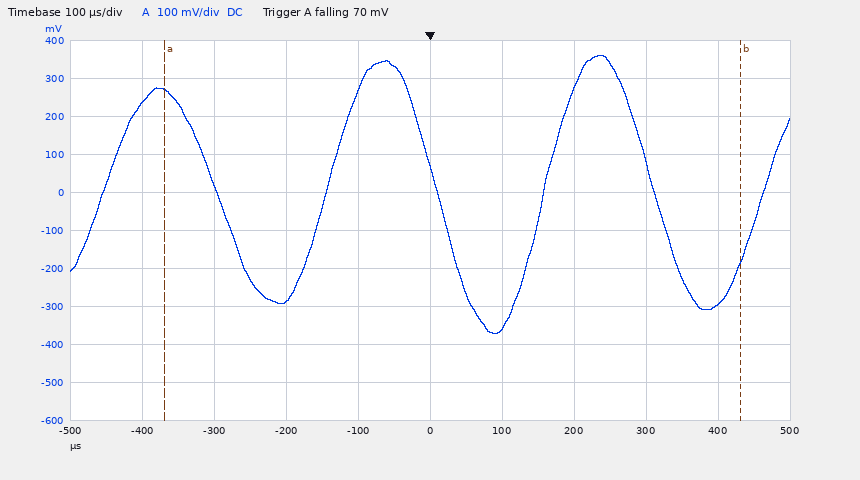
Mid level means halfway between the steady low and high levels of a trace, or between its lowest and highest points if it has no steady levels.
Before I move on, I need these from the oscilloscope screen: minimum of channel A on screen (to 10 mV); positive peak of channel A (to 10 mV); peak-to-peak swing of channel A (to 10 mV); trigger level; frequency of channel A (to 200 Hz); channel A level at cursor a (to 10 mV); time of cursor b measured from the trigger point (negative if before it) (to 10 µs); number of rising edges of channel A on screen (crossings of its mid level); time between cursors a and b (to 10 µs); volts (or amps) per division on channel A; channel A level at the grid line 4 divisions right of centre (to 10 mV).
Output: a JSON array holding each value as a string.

["-370 mV", "360 mV", "730 mV", "70 mV", "3.2 kHz", "270 mV", "+430 µs", "4", "800 µs", "100 mV", "-290 mV"]
